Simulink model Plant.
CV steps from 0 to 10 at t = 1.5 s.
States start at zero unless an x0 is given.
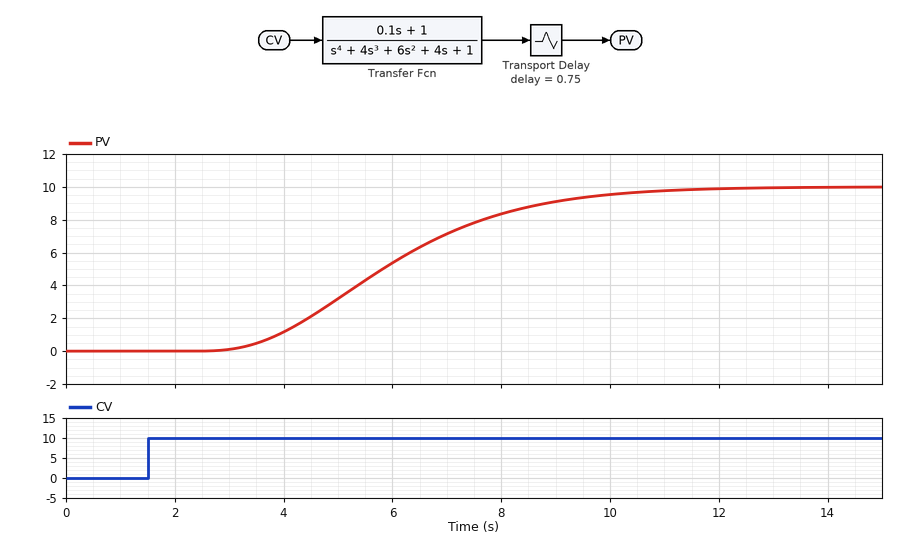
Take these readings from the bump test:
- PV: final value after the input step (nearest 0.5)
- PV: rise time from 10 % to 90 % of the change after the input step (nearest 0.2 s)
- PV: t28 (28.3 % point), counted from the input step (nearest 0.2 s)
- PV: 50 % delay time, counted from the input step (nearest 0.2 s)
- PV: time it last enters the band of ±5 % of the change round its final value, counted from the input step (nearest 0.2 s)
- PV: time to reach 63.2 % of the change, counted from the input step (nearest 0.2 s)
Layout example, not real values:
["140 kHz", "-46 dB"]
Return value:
["10.0", "5.0 s", "3.4 s", "4.4 s", "8.4 s", "5.0 s"]
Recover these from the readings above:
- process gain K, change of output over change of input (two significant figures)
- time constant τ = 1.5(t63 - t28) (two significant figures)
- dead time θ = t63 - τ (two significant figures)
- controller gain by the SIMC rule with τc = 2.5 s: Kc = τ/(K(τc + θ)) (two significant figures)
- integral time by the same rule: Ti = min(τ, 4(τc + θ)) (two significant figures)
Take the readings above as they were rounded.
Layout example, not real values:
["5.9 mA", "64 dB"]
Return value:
["1.0", "2.4 s", "2.6 s", "0.47", "2.4 s"]
